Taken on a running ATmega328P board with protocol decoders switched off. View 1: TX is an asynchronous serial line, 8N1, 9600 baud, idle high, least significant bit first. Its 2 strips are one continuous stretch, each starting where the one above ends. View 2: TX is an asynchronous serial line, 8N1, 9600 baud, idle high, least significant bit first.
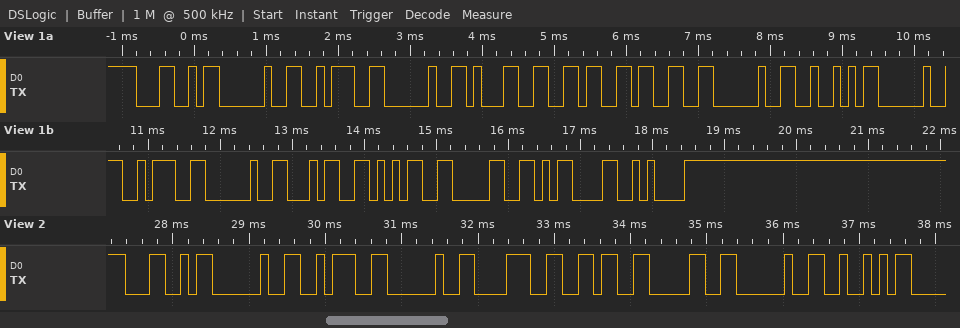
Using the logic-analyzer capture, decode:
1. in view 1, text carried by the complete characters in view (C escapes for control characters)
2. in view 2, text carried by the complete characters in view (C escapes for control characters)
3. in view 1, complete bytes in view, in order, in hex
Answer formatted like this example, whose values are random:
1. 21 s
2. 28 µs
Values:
1. "L : 163 R : 450\r\n"
2. "L : 860 R"
3. 4C 20 3A 20 31 36 33 20 52 20 3A 20 34 35 30 0D 0A
